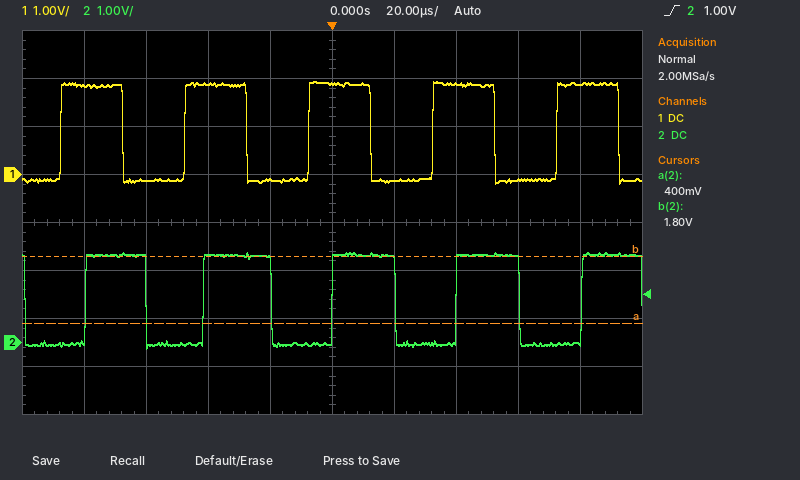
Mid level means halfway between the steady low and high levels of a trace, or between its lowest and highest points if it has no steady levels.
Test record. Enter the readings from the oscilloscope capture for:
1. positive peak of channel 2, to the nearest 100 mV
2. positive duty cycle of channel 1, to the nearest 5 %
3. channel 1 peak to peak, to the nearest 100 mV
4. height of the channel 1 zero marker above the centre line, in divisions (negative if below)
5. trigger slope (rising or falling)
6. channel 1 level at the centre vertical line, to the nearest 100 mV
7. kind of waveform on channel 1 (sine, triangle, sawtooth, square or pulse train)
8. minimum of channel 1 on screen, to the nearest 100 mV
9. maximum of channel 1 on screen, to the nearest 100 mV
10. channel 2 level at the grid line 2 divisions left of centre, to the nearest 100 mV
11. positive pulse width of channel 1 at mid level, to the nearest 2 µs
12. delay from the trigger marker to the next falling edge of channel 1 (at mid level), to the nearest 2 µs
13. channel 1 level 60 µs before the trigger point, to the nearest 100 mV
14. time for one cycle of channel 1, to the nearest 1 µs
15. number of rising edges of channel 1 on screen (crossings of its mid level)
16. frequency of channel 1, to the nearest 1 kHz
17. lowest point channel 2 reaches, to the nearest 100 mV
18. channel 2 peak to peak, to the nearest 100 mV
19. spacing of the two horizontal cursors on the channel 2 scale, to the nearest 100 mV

1.9 V
50 %
2.1 V
+1.0 div
rising
1.9 V
square
-200 mV
1.9 V
1.8 V
20 µs
12 µs
-100 mV
40 µs
5
25 kHz
-100 mV
2.0 V
1.4 V
